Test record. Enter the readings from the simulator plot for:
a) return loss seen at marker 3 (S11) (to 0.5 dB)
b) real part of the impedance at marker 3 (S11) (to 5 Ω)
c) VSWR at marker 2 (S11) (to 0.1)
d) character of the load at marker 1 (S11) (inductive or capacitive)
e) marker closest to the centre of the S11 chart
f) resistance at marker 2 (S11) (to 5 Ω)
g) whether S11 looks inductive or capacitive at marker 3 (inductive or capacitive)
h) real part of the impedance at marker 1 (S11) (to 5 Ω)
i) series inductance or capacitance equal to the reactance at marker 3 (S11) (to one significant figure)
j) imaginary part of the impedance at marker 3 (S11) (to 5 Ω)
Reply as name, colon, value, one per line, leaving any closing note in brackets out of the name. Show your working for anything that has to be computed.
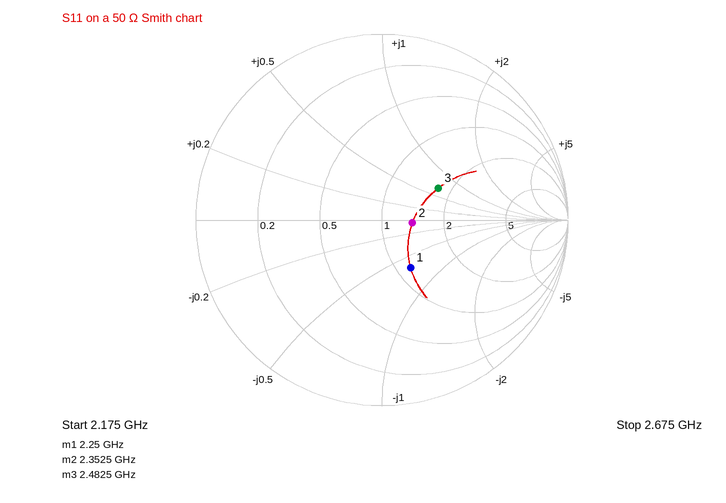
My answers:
return loss seen at marker 3 (S11): 9.0 dB
real part of the impedance at marker 3 (S11): 85 Ω
VSWR at marker 2 (S11): 1.4
character of the load at marker 1 (S11): capacitive
marker closest to the centre of the S11 chart: marker 2
resistance at marker 2 (S11): 70 Ω
whether S11 looks inductive or capacitive at marker 3: inductive
real part of the impedance at marker 1 (S11): 60 Ω
series inductance or capacitance equal to the reactance at marker 3 (S11): L = 35 Ω/(2π × 2.4825 GHz) ≈ 2 nH
imaginary part of the impedance at marker 3 (S11): +35 Ω
